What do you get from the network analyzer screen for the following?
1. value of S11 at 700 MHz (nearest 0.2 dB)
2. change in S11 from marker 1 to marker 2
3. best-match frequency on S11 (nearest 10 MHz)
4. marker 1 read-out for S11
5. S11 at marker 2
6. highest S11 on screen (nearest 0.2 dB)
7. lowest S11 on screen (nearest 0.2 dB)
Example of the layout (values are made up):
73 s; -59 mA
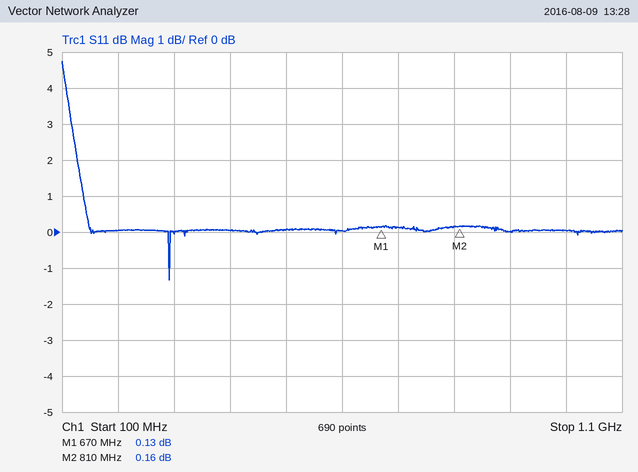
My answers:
0.2 dB; 0.03 dB; 290 MHz; 0.13 dB; 0.16 dB; 4.8 dB; -1.4 dB
